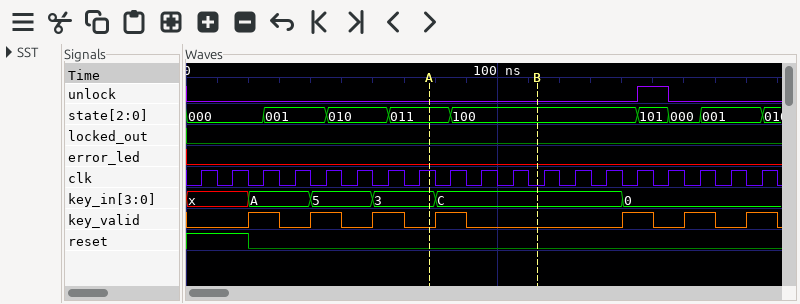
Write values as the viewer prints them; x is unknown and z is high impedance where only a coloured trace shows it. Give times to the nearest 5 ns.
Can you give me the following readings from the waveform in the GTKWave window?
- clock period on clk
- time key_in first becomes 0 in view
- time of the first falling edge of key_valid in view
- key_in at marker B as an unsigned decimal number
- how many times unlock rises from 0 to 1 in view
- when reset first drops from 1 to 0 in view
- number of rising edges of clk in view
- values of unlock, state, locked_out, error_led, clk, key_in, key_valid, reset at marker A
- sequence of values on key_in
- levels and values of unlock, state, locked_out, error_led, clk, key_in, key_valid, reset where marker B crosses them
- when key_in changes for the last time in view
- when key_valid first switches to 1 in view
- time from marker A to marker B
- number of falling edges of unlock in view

10 ns
140 ns
30 ns
12
1
20 ns
19
unlock=0, state=011, locked_out=0, error_led=0, clk=1, key_in=3, key_valid=0, reset=0
x, A, 5, 3, C, 0
unlock=0, state=100, locked_out=0, error_led=0, clk=0, key_in=C, key_valid=0, reset=0
140 ns
20 ns
35 ns
1
